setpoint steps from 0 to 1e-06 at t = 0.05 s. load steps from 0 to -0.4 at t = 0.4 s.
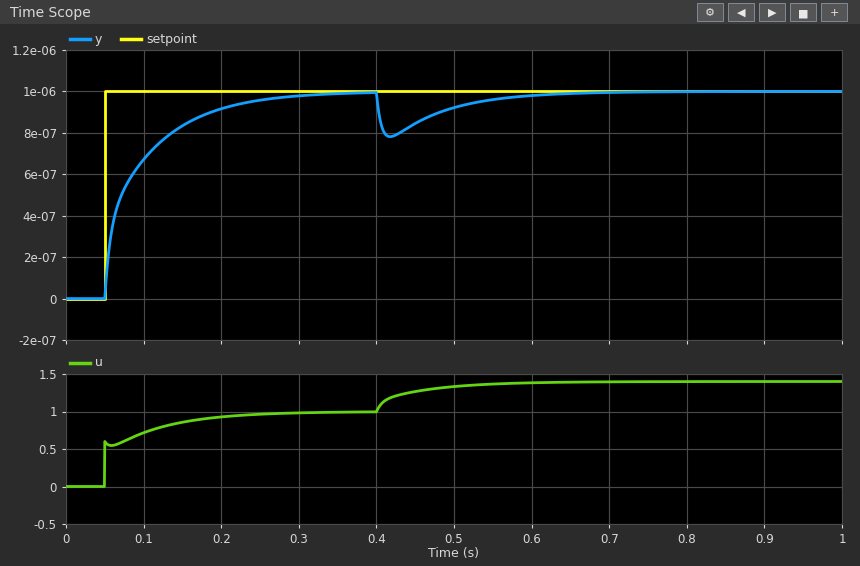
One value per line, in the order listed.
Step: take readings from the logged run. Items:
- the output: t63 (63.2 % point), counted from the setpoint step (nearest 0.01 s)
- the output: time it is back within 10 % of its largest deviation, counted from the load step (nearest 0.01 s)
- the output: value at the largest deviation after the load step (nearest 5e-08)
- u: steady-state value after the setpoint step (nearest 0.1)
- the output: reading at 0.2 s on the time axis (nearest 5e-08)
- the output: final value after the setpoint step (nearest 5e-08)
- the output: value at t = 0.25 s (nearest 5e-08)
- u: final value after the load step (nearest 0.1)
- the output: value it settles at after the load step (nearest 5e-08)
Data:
0.04 s
0.20 s
0.00000080
1.0
0.00000090
0.00000100
0.00000095
1.4
0.00000100
